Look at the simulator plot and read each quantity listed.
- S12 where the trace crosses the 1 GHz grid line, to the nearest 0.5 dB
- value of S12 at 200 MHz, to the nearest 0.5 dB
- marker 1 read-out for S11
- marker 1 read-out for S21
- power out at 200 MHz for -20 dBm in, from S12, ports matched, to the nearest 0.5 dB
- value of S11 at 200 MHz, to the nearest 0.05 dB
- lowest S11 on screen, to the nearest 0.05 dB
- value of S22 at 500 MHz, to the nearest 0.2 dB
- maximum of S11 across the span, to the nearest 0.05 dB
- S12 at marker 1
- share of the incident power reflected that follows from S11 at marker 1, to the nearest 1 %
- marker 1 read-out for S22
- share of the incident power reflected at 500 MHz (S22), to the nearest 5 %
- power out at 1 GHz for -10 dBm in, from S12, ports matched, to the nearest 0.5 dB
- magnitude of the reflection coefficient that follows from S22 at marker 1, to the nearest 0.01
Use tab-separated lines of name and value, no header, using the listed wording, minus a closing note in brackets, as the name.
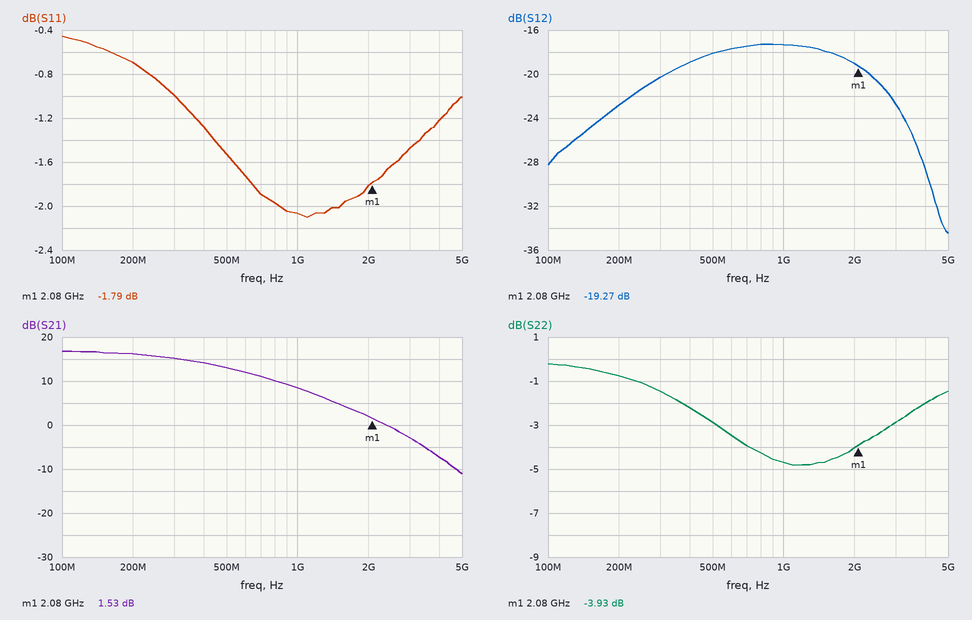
S12 where the trace crosses the 1 GHz grid line, to the nearest 0.5 dB	-17.5 dB
value of S12 at 200 MHz, to the nearest 0.5 dB	-23.0 dB
marker 1 read-out for S11	-1.79 dB
marker 1 read-out for S21	1.53 dB
power out at 200 MHz for -20 dBm in, from S12, ports matched, to the nearest 0.5 dB	-43.0 dBm
value of S11 at 200 MHz, to the nearest 0.05 dB	-0.70 dB
lowest S11 on screen, to the nearest 0.05 dB	-2.10 dB
value of S22 at 500 MHz, to the nearest 0.2 dB	-2.8 dB
maximum of S11 across the span, to the nearest 0.05 dB	-0.45 dB
S12 at marker 1	-19.27 dB
share of the incident power reflected that follows from S11 at marker 1, to the nearest 1 %	66 %
marker 1 read-out for S22	-3.93 dB
share of the incident power reflected at 500 MHz (S22), to the nearest 5 %	50 %
power out at 1 GHz for -10 dBm in, from S12, ports matched, to the nearest 0.5 dB	-27.5 dBm
magnitude of the reflection coefficient that follows from S22 at marker 1, to the nearest 0.01	0.64
